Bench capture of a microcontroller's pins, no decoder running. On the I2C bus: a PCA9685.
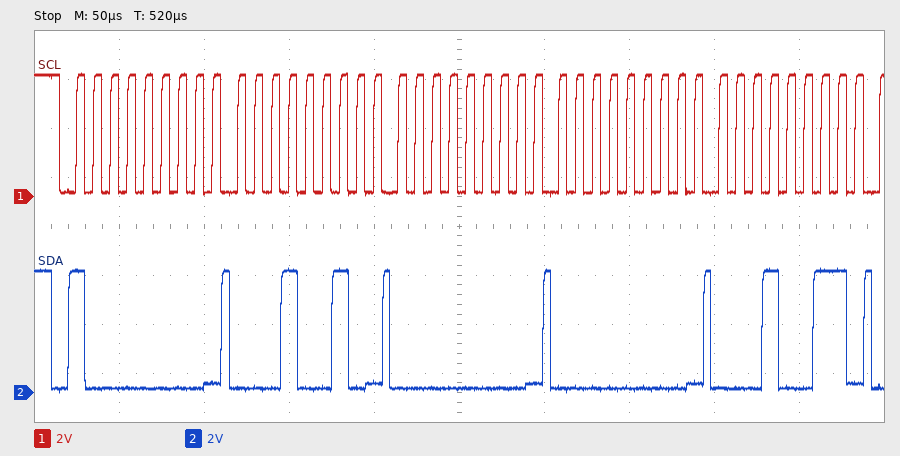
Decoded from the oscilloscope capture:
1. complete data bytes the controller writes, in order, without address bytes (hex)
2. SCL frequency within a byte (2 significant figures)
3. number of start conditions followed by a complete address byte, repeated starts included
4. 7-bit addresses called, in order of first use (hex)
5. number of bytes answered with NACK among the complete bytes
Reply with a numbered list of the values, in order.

1. 12 00 00 13
2. 100 kHz
3. 1
4. 0x40
5. 0
